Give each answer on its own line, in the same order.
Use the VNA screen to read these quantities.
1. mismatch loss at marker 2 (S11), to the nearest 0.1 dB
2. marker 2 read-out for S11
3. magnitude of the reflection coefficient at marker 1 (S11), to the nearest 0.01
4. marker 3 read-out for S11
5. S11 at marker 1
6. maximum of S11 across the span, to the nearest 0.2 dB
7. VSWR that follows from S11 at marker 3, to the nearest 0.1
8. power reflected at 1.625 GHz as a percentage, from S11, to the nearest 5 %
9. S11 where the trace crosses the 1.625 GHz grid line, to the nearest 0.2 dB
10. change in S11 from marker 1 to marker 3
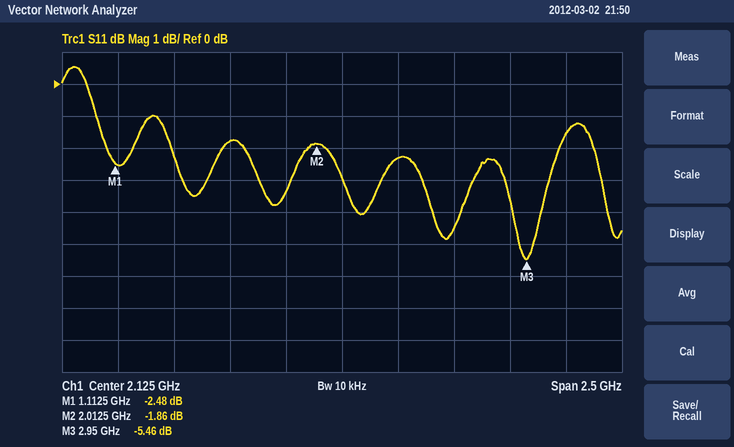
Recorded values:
4.6 dB
-1.86 dB
0.75
-5.46 dB
-2.48 dB
0.6 dB
3.3
65 %
-1.8 dB
-2.98 dB
